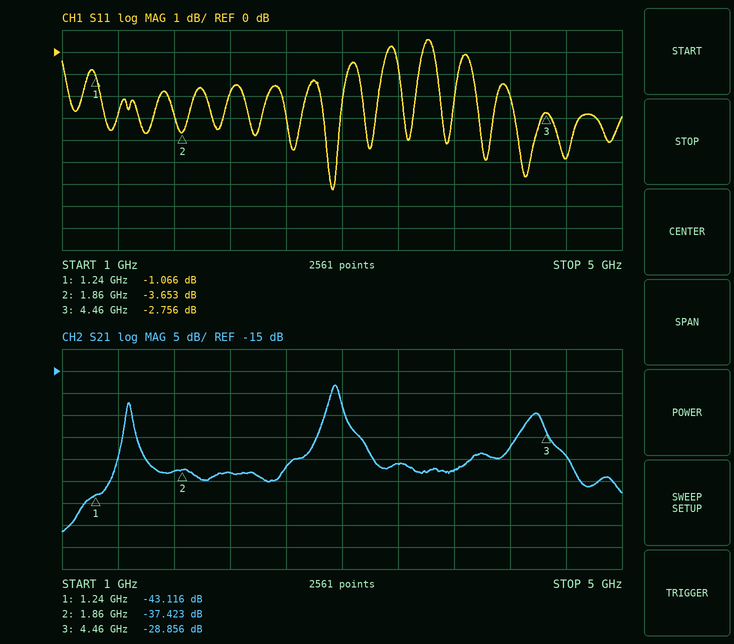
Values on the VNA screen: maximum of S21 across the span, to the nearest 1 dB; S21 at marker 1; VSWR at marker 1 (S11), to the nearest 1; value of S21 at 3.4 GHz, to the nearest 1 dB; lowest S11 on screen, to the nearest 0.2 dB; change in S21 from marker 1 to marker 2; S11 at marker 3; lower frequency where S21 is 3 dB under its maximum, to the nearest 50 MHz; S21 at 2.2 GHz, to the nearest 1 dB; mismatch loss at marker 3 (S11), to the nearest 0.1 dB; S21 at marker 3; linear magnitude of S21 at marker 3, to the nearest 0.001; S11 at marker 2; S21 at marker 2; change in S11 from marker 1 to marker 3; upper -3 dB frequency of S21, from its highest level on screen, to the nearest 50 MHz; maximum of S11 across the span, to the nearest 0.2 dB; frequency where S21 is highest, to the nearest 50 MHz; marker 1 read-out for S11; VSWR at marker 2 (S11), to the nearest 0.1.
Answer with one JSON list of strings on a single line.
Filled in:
["-18 dB", "-43.116 dB", "16", "-36 dB", "-6.2 dB", "5.693 dB", "-2.756 dB", "2.90 GHz", "-38 dB", "3.3 dB", "-28.856 dB", "0.036", "-3.653 dB", "-37.423 dB", "-1.690 dB", "3.00 GHz", "0.6 dB", "2.95 GHz", "-1.066 dB", "4.8"]
